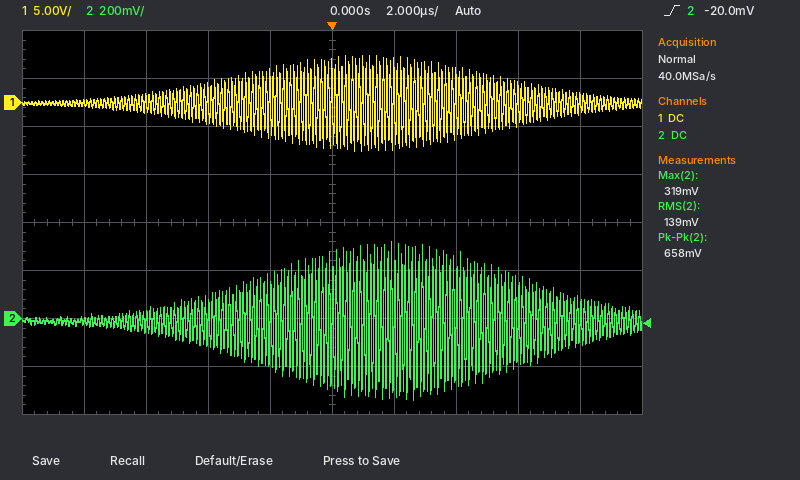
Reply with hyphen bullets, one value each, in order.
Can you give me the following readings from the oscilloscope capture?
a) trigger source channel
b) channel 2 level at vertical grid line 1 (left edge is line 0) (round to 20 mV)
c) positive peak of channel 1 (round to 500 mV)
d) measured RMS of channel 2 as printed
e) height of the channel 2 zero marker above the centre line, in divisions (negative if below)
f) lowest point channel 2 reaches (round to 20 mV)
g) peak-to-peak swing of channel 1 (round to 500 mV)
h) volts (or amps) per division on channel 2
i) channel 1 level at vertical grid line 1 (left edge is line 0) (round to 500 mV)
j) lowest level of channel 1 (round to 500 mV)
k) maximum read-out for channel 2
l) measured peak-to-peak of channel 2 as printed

- channel 2
- 0 mV
- 5.0 V
- 139 mV
- -2.0 div
- -340 mV
- 10.0 V
- 200 mV
- 0.0 V
- -5.0 V
- 319 mV
- 658 mV
